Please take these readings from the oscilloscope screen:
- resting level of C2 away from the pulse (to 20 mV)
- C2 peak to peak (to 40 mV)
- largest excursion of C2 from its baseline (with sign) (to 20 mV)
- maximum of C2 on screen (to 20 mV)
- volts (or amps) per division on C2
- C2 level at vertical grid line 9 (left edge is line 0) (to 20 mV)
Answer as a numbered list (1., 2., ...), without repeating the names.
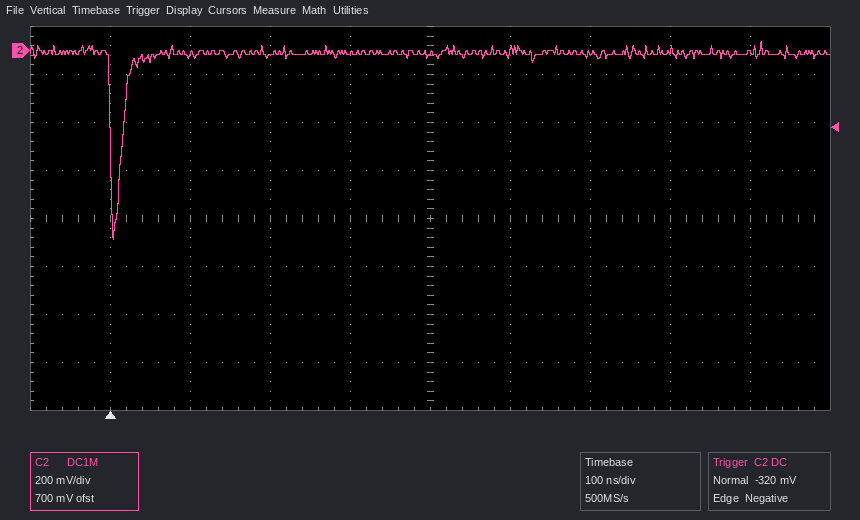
1. -20 mV
2. 840 mV
3. -780 mV
4. 40 mV
5. 200 mV
6. 0 mV
